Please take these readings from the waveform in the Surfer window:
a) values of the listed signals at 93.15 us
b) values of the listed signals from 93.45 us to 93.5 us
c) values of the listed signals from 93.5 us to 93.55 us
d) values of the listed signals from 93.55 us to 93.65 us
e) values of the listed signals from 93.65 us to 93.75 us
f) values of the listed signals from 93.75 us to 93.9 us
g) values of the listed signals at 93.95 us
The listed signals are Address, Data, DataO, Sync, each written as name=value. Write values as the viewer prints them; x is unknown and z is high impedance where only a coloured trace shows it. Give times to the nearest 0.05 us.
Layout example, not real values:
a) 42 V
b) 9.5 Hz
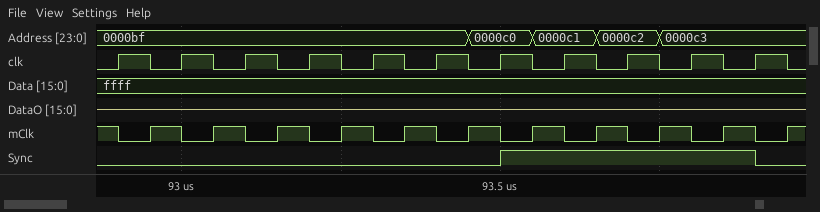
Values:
a) Address=0000bf, Data=ffff, DataO=z, Sync=0
b) Address=0000c0, Data=ffff, DataO=z, Sync=0
c) Address=0000c0, Data=ffff, DataO=z, Sync=1
d) Address=0000c1, Data=ffff, DataO=z, Sync=1
e) Address=0000c2, Data=ffff, DataO=z, Sync=1
f) Address=0000c3, Data=ffff, DataO=z, Sync=1
g) Address=0000c3, Data=ffff, DataO=z, Sync=0
